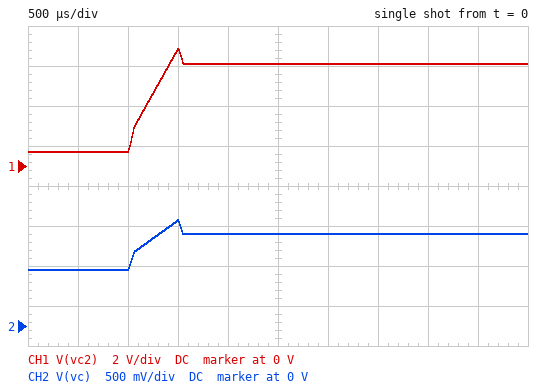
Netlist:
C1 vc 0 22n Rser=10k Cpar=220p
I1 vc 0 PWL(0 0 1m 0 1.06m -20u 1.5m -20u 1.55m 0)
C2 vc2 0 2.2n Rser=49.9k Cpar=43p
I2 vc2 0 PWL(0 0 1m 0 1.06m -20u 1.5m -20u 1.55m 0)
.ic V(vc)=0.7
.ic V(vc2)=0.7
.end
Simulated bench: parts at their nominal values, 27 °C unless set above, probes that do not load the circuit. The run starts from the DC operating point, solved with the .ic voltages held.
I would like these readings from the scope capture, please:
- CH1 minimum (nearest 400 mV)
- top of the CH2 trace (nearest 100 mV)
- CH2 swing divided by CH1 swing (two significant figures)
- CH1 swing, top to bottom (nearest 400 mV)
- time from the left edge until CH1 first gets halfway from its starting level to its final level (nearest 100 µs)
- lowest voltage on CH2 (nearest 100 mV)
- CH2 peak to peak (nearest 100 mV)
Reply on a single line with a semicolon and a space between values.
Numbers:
800 mV; 1.3 V; 0.12; 5.2 V; 1.2 ms; 700 mV; 600 mV
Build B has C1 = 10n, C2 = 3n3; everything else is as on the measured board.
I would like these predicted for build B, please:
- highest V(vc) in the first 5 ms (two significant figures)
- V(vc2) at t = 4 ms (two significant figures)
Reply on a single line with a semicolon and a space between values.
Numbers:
1.8 V; 3.7 V
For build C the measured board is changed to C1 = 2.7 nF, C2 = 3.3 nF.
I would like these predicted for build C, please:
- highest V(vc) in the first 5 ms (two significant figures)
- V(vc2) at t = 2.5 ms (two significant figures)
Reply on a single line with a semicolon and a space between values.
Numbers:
4.1 V; 3.7 V
